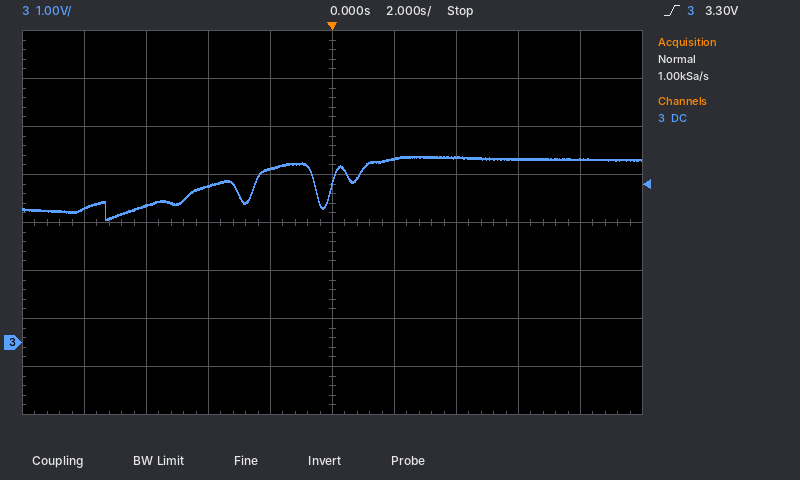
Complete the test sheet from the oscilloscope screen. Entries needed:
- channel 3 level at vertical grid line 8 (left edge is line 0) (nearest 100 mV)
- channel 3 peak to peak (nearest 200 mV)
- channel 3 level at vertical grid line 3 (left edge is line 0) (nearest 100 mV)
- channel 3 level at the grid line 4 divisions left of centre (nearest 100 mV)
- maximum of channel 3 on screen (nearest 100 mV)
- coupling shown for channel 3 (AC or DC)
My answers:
3.8 V
1.4 V
3.3 V
2.8 V
3.9 V
DC
